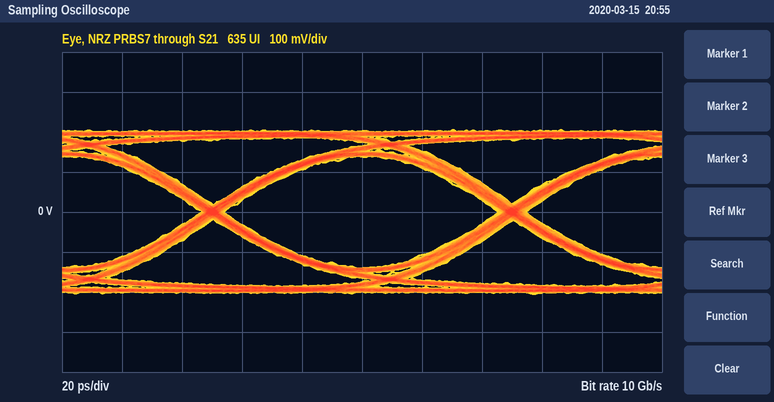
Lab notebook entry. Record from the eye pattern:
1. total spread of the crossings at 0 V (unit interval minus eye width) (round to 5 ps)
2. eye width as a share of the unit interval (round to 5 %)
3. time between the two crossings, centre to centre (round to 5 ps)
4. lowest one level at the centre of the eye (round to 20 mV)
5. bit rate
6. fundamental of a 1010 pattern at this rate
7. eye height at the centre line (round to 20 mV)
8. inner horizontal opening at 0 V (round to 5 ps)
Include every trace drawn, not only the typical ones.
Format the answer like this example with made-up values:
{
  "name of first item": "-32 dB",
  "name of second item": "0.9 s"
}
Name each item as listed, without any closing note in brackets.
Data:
{
  "total spread of the crossings at 0 V (unit interval minus eye width)": "10 ps",
  "eye width as a share of the unit interval": "90 %",
  "time between the two crossings, centre to centre": "100 ps",
  "lowest one level at the centre of the eye": "140 mV",
  "bit rate": "10 Gb/s",
  "fundamental of a 1010 pattern at this rate": "5 GHz",
  "eye height at the centre line": "280 mV",
  "inner horizontal opening at 0 V": "90 ps"
}
